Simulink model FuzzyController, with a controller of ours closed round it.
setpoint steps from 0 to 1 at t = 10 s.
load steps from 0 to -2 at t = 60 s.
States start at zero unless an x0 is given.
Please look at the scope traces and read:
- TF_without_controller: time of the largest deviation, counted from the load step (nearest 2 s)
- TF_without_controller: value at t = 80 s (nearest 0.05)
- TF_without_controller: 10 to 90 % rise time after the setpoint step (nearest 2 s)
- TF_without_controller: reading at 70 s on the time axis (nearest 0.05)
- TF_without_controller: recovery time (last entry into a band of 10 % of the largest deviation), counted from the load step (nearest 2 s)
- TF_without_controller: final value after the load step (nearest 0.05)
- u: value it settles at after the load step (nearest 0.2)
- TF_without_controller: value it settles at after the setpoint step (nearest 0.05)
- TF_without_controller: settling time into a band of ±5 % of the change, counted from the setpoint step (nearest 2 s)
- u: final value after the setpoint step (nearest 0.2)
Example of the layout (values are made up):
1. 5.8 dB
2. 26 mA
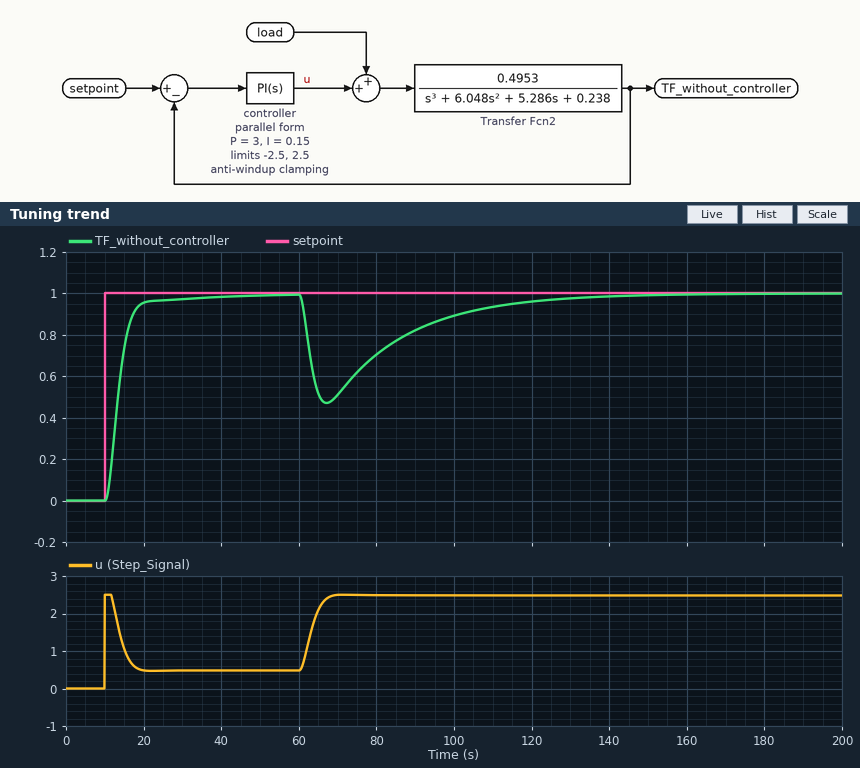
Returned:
1. 8 s
2. 0.70
3. 6 s
4. 0.50
5. 54 s
6. 1.00
7. 2.4
8. 1.00
9. 10 s
10. 0.4
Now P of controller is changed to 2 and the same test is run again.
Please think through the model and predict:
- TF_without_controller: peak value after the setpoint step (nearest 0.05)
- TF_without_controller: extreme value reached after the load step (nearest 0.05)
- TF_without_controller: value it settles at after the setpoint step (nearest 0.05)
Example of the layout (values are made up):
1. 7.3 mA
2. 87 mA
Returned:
1. 1.05
2. 0.35
3. 1.00
